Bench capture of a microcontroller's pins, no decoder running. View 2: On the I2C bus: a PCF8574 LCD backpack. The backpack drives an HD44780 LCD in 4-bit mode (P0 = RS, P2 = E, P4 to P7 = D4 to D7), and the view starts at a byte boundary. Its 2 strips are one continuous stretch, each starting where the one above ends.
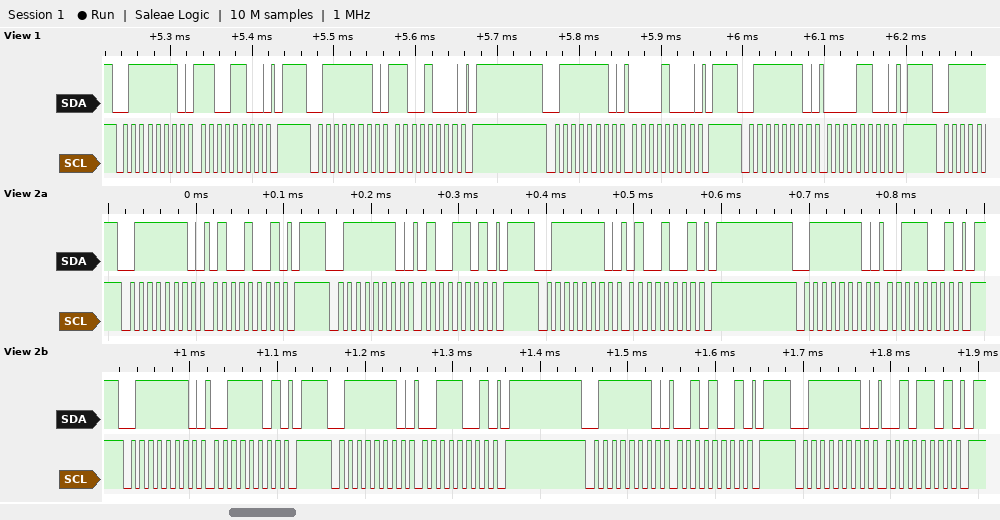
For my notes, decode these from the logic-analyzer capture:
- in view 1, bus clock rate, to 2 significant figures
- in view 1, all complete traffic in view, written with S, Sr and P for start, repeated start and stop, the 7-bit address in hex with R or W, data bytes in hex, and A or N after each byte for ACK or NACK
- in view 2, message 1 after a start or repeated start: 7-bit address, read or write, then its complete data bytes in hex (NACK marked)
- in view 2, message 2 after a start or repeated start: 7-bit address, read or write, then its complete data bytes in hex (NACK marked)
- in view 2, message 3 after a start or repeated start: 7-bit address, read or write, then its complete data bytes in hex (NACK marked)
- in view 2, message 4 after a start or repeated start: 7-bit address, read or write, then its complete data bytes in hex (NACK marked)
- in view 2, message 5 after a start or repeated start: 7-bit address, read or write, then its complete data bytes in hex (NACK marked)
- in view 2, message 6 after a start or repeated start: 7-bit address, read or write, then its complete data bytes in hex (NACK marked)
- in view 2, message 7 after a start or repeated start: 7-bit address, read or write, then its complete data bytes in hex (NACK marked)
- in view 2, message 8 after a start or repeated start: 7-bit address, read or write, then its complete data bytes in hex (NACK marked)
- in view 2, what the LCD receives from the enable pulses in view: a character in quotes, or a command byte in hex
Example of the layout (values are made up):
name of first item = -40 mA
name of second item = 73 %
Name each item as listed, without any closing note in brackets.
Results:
in view 1, bus clock rate, to 2 significant figures = 100 kHz
in view 1, all complete traffic in view, written with S, Sr and P for start, repeated start and stop, the 7-bit address in hex with R or W, data bytes in hex, and A or N after each byte for ACK or NACK = S 3FW A CC A P S 3FW A C8 A P S 3FW A 08 A P S 3FW A 0C A P
in view 2, message 1 after a start or repeated start: 7-bit address, read or write, then its complete data bytes in hex = 0x3F write: 49
in view 2, message 2 after a start or repeated start: 7-bit address, read or write, then its complete data bytes in hex = 0x3F write: 4D
in view 2, message 3 after a start or repeated start: 7-bit address, read or write, then its complete data bytes in hex = 0x3F write: 49
in view 2, message 4 after a start or repeated start: 7-bit address, read or write, then its complete data bytes in hex = 0x3F write: 39
in view 2, message 5 after a start or repeated start: 7-bit address, read or write, then its complete data bytes in hex = 0x3F write: 3D
in view 2, message 6 after a start or repeated start: 7-bit address, read or write, then its complete data bytes in hex = 0x3F write: 39
in view 2, message 7 after a start or repeated start: 7-bit address, read or write, then its complete data bytes in hex = 0x3F write: 29
in view 2, message 8 after a start or repeated start: 7-bit address, read or write, then its complete data bytes in hex = 0x3F write: 2D
in view 2, what the LCD receives from the enable pulses in view: a character in quotes, or a command byte in hex = 'C'
